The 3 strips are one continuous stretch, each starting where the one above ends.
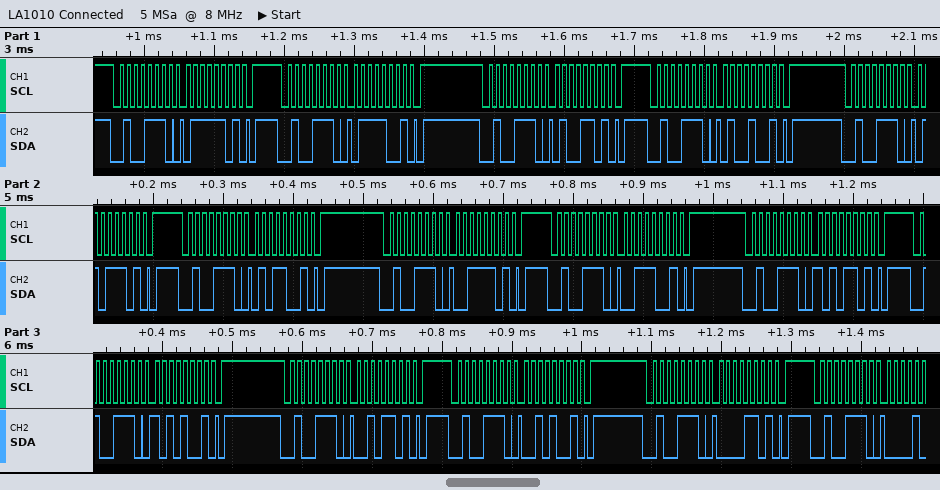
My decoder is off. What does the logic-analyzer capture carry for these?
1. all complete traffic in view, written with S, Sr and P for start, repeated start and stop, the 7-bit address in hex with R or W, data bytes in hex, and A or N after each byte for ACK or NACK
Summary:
S 27W A 7D A P S 27W A 79 A P S 27W A 4D A P S 27W A 49 A P S 27W A 5D A P S 27W A 59 A P S 27W A 3D A P S 27W A 39 A P S 27W A AD A P S 27W A A9 A P S 27W A 2D A P S 27W A 29 A P S 27W A 0D A P S 27W A
